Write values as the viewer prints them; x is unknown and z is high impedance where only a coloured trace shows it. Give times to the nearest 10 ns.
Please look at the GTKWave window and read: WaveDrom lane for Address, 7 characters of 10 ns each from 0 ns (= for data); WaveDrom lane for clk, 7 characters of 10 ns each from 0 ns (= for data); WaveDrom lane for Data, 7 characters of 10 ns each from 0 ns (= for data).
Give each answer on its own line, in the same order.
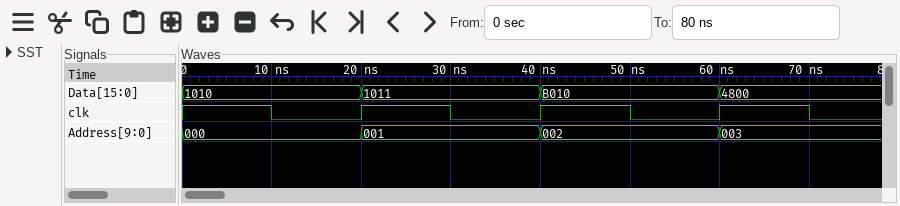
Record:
{name: 'Address', wave: '=.=.=.=', data: '000 001 002 003'}
{name: 'clk', wave: '1010101'}
{name: 'Data', wave: '=.=.=.=', data: '1010 1011 B010 4800'}
